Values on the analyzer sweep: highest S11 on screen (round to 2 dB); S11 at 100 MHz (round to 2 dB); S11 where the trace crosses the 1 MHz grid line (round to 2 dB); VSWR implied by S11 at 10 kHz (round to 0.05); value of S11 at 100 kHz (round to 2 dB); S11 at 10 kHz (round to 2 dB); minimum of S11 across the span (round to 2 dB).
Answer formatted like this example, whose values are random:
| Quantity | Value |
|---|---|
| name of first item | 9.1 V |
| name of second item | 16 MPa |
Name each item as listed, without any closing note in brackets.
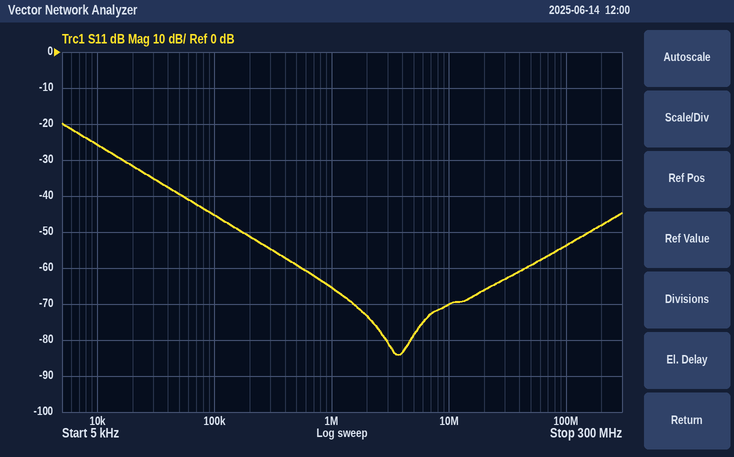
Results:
| Quantity | Value |
|---|---|
| highest S11 on screen | -20 dB |
| S11 at 100 MHz | -54 dB |
| S11 where the trace crosses the 1 MHz grid line | -66 dB |
| VSWR implied by S11 at 10 kHz | 1.10 |
| value of S11 at 100 kHz | -46 dB |
| S11 at 10 kHz | -26 dB |
| minimum of S11 across the span | -84 dB |
